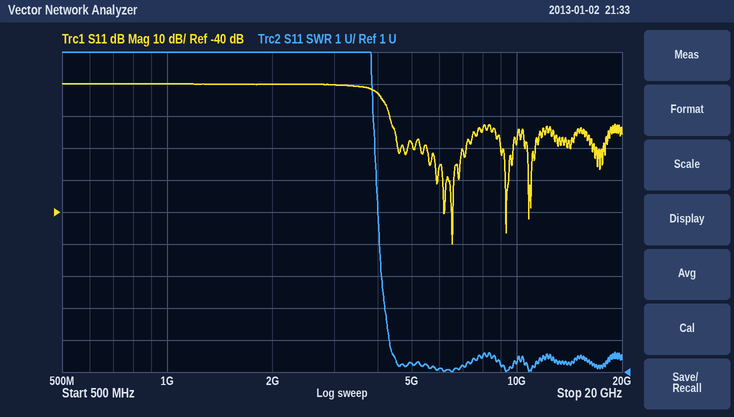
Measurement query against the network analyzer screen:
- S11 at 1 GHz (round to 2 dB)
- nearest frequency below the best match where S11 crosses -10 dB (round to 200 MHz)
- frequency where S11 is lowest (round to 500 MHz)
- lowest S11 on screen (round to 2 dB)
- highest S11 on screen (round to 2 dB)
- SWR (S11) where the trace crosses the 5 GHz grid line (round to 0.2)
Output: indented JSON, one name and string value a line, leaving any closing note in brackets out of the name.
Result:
{
  "S11 at 1 GHz": "0 dB",
  "nearest frequency below the best match where S11 crosses -10 dB": "4.4 GHz",
  "frequency where S11 is lowest": "6.5 GHz",
  "lowest S11 on screen": "-50 dB",
  "highest S11 on screen": "0 dB",
  "SWR (S11) where the trace crosses the 5 GHz grid line": "1.2"
}
